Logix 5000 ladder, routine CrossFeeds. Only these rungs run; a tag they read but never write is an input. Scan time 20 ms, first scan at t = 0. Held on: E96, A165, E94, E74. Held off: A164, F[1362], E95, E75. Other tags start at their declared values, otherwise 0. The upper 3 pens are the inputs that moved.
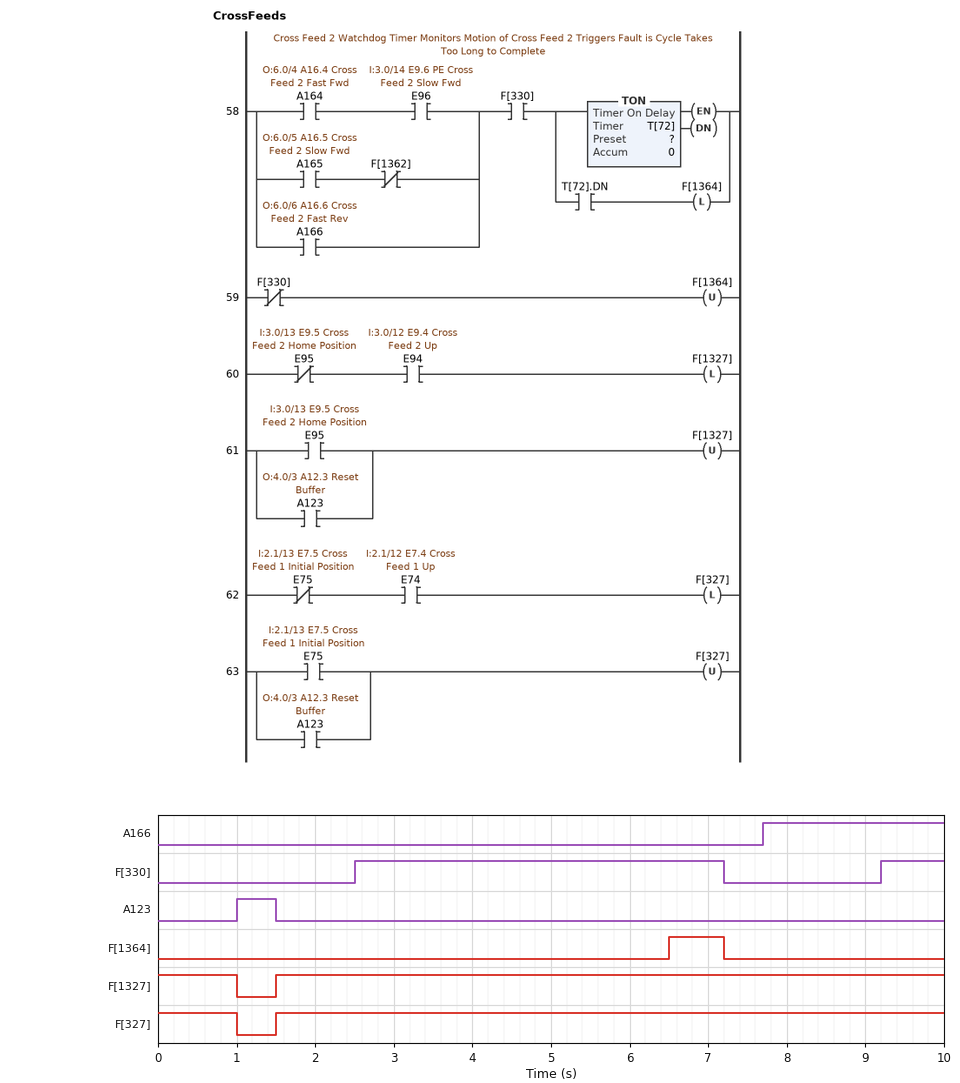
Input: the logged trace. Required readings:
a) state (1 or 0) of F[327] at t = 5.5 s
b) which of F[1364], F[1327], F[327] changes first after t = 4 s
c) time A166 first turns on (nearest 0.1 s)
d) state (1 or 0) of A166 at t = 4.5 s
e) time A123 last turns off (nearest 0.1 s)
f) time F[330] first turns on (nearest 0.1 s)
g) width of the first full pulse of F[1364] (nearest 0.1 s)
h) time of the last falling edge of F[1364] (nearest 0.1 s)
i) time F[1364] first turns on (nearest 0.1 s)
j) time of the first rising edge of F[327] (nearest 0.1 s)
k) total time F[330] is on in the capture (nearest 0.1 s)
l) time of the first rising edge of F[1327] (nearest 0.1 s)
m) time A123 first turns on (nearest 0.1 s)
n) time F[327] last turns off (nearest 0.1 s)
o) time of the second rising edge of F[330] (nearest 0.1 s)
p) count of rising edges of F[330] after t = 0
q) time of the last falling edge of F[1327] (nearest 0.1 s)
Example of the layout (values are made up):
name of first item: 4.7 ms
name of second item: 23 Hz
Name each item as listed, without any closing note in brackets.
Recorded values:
state (1 or 0) of F[327] at t = 5.5 s: 1
which of F[1364], F[1327], F[327] changes first after t = 4 s: F[1364]
time A166 first turns on: 7.7 s
state (1 or 0) of A166 at t = 4.5 s: 0
time A123 last turns off: 1.5 s
time F[330] first turns on: 2.5 s
width of the first full pulse of F[1364]: 0.7 s
time of the last falling edge of F[1364]: 7.2 s
time F[1364] first turns on: 6.5 s
time of the first rising edge of F[327]: 1.5 s
total time F[330] is on in the capture: 5.5 s
time of the first rising edge of F[1327]: 1.5 s
time A123 first turns on: 1.0 s
time F[327] last turns off: 1.0 s
time of the second rising edge of F[330]: 9.2 s
count of rising edges of F[330] after t = 0: 2
time of the last falling edge of F[1327]: 1.0 s
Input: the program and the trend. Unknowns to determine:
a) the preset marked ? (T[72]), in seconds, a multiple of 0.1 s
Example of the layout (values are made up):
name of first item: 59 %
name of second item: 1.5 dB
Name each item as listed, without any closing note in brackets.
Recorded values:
the preset marked ? (T[72]), in seconds, a multiple of 0.1 s: 4.0 s
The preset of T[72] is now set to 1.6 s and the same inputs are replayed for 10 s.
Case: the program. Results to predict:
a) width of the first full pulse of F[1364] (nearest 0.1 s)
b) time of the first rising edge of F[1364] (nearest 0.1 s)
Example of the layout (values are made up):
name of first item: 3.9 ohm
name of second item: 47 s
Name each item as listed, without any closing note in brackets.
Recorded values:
width of the first full pulse of F[1364]: 3.1 s
time of the first rising edge of F[1364]: 4.1 s
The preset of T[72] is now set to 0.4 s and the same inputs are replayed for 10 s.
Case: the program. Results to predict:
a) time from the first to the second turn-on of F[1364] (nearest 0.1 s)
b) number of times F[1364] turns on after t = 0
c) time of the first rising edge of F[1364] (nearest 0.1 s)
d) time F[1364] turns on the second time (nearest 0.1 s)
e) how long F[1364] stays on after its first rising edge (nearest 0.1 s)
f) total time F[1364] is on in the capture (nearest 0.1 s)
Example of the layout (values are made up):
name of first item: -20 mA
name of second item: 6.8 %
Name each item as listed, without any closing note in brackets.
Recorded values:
time from the first to the second turn-on of F[1364]: 6.7 s
number of times F[1364] turns on after t = 0: 2
time of the first rising edge of F[1364]: 2.9 s
time F[1364] turns on the second time: 9.6 s
how long F[1364] stays on after its first rising edge: 4.3 s
total time F[1364] is on in the capture: 4.7 s
